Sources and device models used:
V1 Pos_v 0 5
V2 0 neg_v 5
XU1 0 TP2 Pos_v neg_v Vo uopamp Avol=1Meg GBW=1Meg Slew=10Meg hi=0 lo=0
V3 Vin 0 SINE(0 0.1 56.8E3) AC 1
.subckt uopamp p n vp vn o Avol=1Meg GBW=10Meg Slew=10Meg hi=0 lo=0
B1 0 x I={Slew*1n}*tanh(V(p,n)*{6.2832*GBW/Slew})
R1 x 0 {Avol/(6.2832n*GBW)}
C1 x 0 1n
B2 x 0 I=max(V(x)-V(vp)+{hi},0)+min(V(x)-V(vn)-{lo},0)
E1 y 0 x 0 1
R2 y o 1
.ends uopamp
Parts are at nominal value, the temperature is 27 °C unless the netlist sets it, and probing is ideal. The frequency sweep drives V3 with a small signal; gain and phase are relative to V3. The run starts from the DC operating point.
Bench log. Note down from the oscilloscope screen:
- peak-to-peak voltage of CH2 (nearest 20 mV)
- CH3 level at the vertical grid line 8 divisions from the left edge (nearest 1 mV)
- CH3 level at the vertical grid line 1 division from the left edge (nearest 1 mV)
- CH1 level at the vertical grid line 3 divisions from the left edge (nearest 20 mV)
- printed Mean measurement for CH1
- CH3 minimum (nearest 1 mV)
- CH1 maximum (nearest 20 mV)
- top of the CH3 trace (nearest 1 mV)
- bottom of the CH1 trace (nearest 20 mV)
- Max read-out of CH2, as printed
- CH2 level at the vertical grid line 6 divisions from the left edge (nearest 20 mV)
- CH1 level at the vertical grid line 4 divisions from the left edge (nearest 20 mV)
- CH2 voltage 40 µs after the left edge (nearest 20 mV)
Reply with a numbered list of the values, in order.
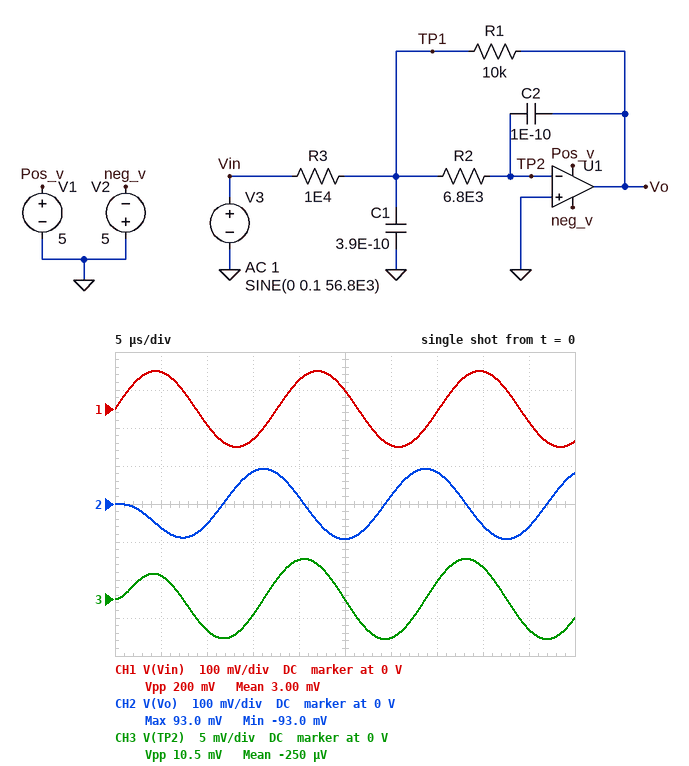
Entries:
1. 180 mV
2. 4 mV
3. 3 mV
4. -80 mV
5. 3.00 mV
6. -5 mV
7. 100 mV
8. 5 mV
9. -100 mV
10. 93.0 mV
11. 20 mV
12. 80 mV
13. -60 mV
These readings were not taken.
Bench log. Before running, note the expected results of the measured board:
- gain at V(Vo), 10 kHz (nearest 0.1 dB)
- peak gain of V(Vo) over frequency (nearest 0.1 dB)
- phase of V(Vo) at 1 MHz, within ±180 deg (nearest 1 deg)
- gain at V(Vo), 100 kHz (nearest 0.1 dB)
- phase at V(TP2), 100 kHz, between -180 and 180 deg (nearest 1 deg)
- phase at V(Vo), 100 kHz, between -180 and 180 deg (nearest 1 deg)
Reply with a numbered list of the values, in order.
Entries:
1. 0 dB
2. 0 dB
3. -32 deg
4. -4.3 dB
5. -16 deg
6. 74 deg
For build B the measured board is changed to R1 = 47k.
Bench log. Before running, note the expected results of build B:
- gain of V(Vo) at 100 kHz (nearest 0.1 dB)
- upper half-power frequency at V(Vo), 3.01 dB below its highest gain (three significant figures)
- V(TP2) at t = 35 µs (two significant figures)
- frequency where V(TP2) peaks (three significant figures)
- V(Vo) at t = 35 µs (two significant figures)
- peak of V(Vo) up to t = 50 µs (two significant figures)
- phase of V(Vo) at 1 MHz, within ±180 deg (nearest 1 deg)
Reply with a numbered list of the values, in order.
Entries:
1. -4.4 dB
2. 20.5 kHz
3. -3.1 mV
4. 40.3 kHz
5. 120 mV
6. 130 mV
7. -33 deg
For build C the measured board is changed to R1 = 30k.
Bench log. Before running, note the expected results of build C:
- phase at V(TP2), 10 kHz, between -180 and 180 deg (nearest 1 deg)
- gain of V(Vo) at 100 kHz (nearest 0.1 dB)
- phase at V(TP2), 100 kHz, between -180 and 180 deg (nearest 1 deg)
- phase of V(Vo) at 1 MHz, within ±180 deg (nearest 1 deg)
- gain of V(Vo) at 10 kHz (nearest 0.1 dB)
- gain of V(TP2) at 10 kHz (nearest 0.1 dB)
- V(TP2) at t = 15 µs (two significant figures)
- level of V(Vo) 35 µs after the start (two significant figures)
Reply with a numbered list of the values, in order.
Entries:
1. 67 deg
2. -4.3 dB
3. -41 deg
4. -33 deg
5. 9.2 dB
6. -30.8 dB
7. -7.1 mV
8. 130 mV
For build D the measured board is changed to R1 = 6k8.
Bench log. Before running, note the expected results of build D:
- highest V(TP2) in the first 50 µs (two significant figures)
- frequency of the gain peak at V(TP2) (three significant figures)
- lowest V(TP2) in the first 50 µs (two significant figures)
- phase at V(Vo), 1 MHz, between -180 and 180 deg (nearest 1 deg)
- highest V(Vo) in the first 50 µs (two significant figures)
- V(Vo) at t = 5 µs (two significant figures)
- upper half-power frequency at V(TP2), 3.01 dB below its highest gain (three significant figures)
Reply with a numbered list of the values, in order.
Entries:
1. 3.9 mV
2. 105 kHz
3. -3.9 mV
4. -31 deg
5. 68 mV
6. -52 mV
7. 193 kHz
